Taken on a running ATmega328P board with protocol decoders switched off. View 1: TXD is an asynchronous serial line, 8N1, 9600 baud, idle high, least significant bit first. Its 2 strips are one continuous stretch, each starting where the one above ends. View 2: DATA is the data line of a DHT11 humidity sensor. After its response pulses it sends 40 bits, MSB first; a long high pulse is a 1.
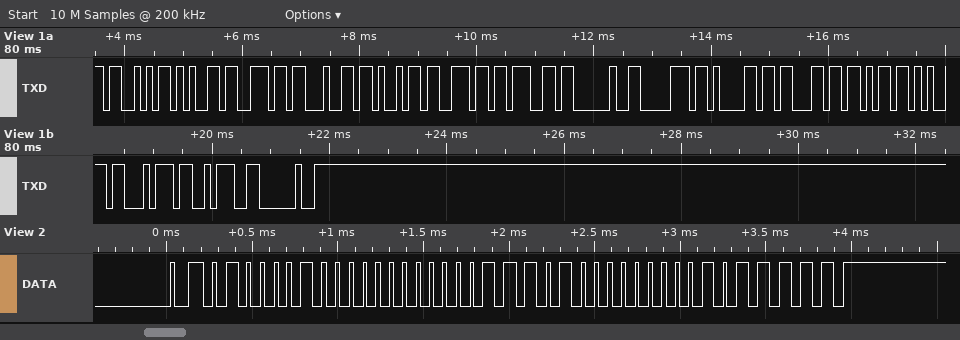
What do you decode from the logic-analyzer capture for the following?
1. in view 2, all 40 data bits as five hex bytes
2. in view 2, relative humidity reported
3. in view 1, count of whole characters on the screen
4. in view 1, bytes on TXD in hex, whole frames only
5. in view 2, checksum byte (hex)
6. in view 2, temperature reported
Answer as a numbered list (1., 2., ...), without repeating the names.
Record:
1. 42 00 1D 00 5F
2. 66 %
3. 16
4. 0x53 0x65 0x6E 0x64 0x69 0x6E 0x67 0x20 0x70 0x61 0x63 0x6B 0x65 0x74 0x3A 0x20
5. 0x5F
6. 29.0 °C
